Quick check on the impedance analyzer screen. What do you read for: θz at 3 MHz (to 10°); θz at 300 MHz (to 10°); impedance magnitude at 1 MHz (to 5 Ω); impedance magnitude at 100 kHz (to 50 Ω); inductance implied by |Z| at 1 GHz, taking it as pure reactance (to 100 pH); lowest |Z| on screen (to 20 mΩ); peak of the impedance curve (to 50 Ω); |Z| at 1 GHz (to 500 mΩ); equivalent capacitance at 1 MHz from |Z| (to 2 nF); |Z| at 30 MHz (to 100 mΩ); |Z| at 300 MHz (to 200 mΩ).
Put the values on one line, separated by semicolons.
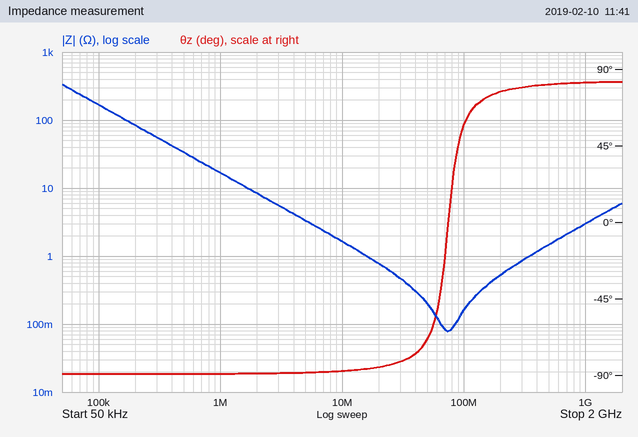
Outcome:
-90°; 80°; 15 Ω; 150 Ω; 500 pH; 80 mΩ; 350 Ω; 3.0 Ω; 10 nF; 500 mΩ; 800 mΩ
